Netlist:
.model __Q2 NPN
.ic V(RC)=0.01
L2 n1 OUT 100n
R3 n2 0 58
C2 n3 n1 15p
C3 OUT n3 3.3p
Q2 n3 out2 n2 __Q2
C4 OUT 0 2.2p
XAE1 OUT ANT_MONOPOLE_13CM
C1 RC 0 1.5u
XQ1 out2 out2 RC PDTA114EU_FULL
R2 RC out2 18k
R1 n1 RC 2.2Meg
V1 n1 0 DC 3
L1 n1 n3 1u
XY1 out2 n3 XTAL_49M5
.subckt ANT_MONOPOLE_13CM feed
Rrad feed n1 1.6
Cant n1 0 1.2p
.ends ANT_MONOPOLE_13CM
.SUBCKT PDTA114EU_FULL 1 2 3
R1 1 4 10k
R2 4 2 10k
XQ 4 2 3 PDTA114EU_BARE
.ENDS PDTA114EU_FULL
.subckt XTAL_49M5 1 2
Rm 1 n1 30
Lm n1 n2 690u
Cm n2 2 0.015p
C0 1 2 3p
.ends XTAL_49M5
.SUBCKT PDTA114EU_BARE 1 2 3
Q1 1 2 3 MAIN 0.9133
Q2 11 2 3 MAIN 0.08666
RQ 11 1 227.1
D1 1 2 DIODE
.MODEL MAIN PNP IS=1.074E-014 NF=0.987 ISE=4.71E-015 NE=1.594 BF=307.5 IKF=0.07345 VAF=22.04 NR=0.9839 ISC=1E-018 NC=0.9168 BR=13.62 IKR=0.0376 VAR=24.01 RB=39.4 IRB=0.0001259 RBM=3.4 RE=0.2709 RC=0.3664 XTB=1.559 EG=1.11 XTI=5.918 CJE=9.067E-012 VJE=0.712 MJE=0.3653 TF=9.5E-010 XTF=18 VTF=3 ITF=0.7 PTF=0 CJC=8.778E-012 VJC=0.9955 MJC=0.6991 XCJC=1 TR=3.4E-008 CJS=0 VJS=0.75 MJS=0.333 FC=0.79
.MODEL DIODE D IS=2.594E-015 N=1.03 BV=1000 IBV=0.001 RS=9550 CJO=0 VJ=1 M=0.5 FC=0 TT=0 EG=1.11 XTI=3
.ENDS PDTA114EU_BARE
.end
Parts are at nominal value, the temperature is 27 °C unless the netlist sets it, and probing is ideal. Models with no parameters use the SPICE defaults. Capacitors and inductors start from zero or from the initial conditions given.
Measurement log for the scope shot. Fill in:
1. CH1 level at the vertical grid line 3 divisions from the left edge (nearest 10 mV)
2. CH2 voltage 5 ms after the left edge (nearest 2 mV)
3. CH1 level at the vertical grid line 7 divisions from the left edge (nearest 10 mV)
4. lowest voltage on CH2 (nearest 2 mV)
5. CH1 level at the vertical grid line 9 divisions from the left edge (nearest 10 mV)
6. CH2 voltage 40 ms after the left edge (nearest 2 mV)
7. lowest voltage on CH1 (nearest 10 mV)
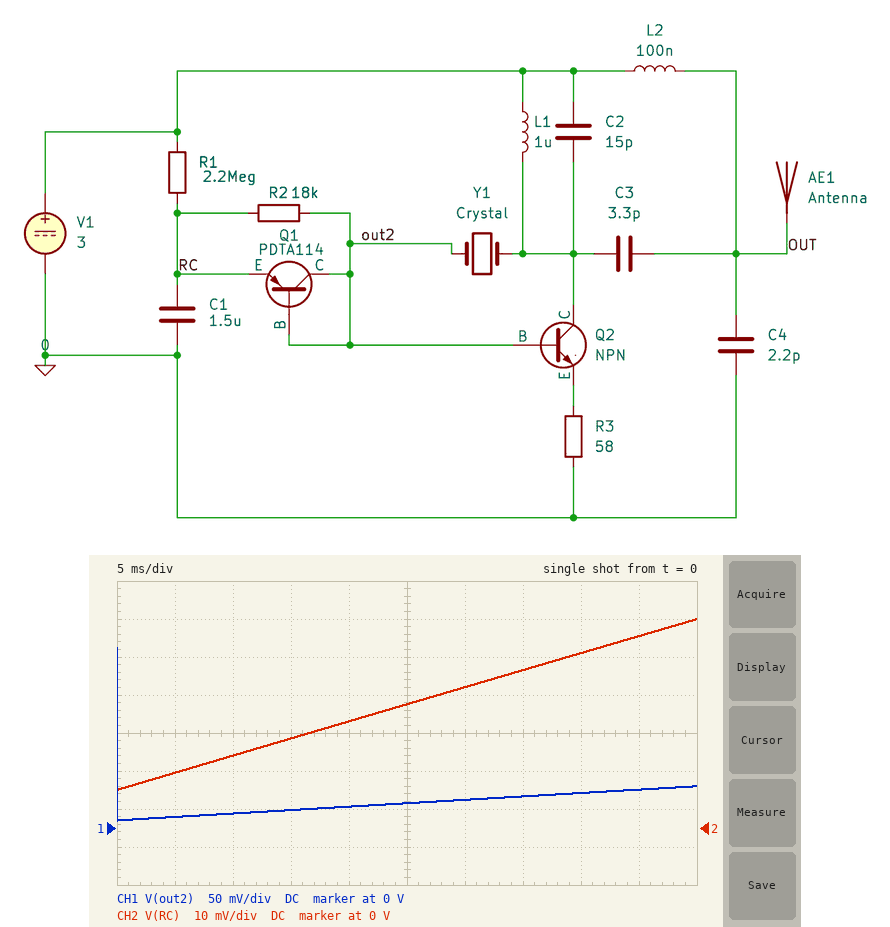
20 mV
14 mV
40 mV
10 mV
50 mV
46 mV
10 mV
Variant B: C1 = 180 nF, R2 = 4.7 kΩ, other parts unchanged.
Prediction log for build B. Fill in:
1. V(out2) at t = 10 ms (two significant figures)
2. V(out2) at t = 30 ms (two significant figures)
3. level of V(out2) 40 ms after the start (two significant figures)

85 mV
230 mV
300 mV
